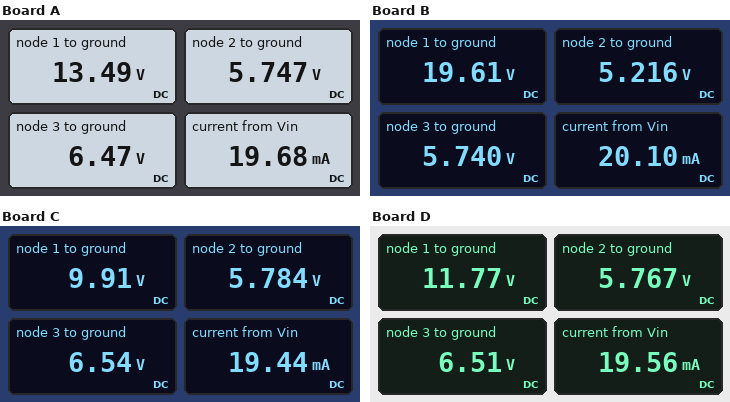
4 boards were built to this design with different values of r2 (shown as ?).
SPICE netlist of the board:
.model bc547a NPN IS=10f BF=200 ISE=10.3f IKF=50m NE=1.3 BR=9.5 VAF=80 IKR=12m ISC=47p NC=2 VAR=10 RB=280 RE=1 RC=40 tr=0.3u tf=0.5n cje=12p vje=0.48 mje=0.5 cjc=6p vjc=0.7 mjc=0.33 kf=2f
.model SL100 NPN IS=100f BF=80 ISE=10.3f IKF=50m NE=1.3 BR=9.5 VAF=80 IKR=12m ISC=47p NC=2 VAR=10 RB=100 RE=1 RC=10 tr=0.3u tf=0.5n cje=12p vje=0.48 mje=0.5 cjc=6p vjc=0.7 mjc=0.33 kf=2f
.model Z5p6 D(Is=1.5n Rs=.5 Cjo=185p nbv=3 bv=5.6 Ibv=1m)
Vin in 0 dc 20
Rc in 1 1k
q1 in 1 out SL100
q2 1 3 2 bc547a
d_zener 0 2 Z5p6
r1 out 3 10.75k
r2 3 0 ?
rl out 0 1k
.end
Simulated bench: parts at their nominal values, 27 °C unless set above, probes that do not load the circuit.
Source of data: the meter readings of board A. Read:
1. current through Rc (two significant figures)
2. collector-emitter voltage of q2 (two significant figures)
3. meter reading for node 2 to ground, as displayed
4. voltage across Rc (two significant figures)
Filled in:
6.5 mA
7.7 V
5.747 V
6.5 V
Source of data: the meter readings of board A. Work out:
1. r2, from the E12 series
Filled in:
12 kΩ
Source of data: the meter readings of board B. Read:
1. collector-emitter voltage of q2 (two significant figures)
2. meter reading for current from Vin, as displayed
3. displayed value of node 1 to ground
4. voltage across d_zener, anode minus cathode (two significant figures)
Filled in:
14 V
20.10 mA
19.61 V
-5.2 V
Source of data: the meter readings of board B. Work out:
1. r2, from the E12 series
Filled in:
4.7 kΩ
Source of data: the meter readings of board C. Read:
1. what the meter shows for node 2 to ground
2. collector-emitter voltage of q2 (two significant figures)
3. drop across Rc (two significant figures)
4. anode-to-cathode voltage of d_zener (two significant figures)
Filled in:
5.784 V
4.1 V
10 V
-5.8 V
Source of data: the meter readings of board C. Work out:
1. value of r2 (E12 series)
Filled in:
39 kΩ
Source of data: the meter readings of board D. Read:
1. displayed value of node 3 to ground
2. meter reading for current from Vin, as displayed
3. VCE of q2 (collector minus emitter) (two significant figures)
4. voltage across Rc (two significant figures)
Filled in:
6.51 V
19.56 mA
6.0 V
8.2 V
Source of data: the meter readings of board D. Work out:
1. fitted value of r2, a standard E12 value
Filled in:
18 kΩ
